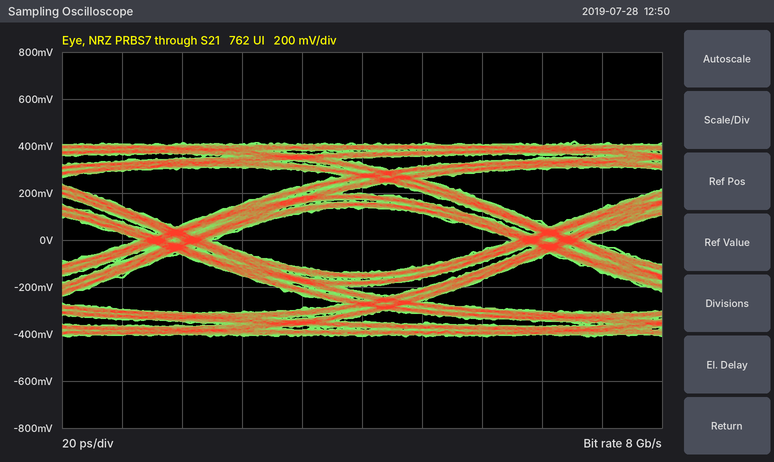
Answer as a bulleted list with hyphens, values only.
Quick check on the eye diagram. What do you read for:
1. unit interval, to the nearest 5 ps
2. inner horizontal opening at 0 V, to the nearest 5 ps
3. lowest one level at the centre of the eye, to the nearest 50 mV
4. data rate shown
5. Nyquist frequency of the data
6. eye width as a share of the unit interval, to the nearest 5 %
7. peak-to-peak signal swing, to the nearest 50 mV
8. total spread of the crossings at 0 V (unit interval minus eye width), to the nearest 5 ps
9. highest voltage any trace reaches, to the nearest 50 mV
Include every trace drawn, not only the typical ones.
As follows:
- 125 ps
- 100 ps
- 150 mV
- 8 Gb/s
- 4 GHz
- 80 %
- 850 mV
- 25 ps
- 400 mV
